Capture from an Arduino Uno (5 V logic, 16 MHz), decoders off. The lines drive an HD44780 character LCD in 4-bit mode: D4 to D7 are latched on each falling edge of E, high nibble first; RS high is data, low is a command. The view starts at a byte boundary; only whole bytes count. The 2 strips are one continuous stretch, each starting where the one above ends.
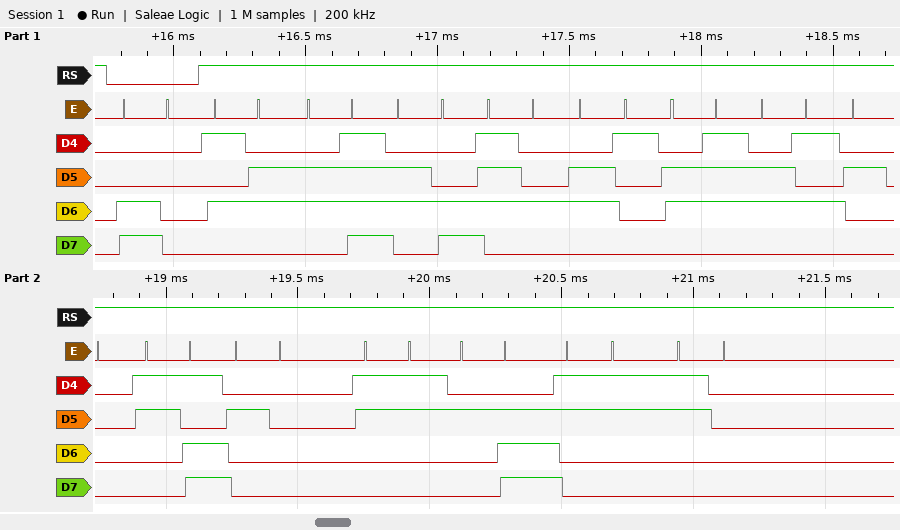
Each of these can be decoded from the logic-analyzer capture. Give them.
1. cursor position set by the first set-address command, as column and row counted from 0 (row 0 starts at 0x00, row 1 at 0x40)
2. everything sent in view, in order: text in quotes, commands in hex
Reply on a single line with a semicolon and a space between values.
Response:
column 0, row 1; 0xC0 "Voltage = 3.30"
